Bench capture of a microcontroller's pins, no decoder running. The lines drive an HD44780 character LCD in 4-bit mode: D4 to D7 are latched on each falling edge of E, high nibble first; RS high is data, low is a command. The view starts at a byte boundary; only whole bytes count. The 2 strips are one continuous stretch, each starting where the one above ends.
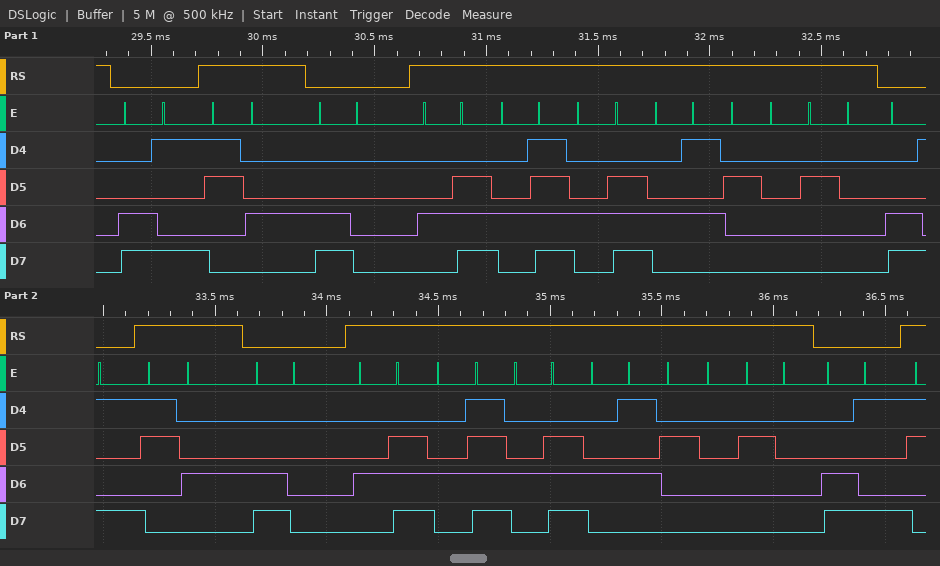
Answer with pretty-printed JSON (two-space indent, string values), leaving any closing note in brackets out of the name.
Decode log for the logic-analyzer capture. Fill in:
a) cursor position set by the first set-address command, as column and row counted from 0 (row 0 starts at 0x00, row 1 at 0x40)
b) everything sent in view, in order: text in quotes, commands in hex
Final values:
{
  "cursor position set by the first set-address command, as column and row counted from 0": "column 9, row 1",
  "everything sent in view, in order: text in quotes, commands in hex": "0xC9 \"4\" 0xC0 \"NONE  \" 0xC9 \"4\" 0xC0 \"NONE  \" 0xC9"
}
